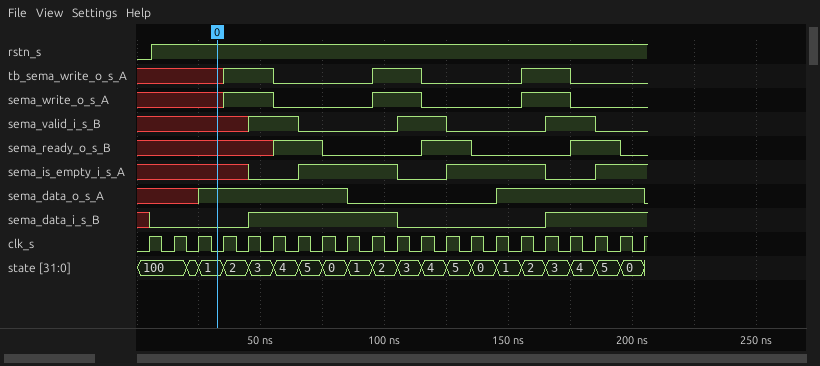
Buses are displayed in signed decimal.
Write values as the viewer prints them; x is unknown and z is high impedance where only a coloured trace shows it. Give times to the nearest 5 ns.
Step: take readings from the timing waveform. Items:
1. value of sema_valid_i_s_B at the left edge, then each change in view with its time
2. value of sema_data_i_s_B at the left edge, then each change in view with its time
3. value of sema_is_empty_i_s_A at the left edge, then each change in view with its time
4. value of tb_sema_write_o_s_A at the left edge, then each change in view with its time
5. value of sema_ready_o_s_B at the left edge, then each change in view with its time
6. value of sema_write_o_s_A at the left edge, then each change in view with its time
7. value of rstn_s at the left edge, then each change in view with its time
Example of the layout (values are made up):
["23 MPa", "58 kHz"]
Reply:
["x, 1 at 45 ns, 0 at 65 ns, 1 at 105 ns, 0 at 125 ns, 1 at 165 ns, 0 at 185 ns", "x, 0 at 5 ns, 1 at 45 ns, 0 at 105 ns, 1 at 165 ns", "x, 0 at 45 ns, 1 at 65 ns, 0 at 105 ns, 1 at 125 ns, 0 at 165 ns, 1 at 185 ns", "x, 1 at 35 ns, 0 at 55 ns, 1 at 95 ns, 0 at 115 ns, 1 at 155 ns, 0 at 175 ns", "x, 1 at 55 ns, 0 at 75 ns, 1 at 115 ns, 0 at 135 ns, 1 at 175 ns, 0 at 195 ns", "x, 1 at 35 ns, 0 at 55 ns, 1 at 95 ns, 0 at 115 ns, 1 at 155 ns, 0 at 175 ns", "0, 1 at 5 ns"]
